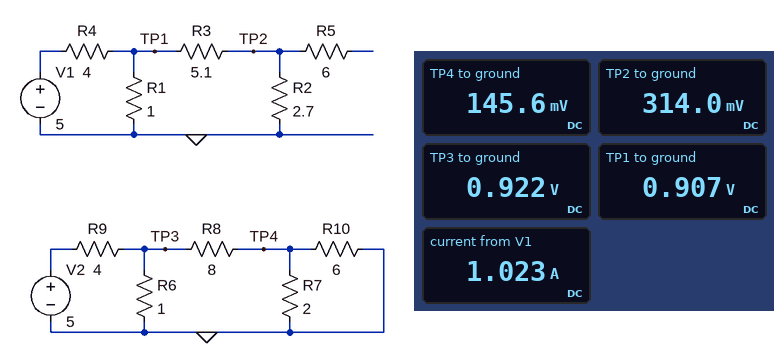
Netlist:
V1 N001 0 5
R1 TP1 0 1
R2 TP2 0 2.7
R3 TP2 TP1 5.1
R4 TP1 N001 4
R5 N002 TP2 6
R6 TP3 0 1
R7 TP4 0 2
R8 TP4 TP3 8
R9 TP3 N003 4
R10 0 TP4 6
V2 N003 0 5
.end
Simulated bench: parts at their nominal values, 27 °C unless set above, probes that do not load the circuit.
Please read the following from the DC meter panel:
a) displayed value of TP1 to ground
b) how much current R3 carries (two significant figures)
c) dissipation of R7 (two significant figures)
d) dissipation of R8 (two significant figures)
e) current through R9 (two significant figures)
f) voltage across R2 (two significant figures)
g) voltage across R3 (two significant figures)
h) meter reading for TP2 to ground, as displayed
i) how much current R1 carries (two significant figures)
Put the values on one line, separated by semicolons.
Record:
0.907 V; 120 mA; 11 mW; 75 mW; 1.0 A; 310 mV; 590 mV; 314.0 mV; 910 mA
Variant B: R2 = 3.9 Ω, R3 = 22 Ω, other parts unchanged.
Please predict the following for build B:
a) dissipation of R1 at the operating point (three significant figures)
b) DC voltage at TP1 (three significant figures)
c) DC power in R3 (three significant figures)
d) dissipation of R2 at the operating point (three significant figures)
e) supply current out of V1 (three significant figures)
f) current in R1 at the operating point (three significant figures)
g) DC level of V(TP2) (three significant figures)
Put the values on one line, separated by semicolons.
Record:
941 mW; 970 mV; 30.9 mW; 5.47 mW; 1.01 A; 970 mA; 146 mV
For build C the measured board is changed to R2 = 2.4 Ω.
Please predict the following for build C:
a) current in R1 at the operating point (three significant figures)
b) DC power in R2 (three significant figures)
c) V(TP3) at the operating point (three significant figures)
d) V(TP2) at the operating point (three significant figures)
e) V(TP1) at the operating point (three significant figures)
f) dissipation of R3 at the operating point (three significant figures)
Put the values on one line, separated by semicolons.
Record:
904 mA; 34.8 mW; 922 mV; 289 mV; 904 mV; 74.0 mW
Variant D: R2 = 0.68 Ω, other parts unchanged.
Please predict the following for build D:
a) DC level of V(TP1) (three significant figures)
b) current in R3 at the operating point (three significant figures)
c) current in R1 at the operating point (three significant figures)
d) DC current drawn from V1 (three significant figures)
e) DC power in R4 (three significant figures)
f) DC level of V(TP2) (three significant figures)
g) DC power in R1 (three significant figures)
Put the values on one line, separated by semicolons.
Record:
878 mV; 152 mA; 878 mA; 1.03 A; 4.25 W; 103 mV; 772 mW
